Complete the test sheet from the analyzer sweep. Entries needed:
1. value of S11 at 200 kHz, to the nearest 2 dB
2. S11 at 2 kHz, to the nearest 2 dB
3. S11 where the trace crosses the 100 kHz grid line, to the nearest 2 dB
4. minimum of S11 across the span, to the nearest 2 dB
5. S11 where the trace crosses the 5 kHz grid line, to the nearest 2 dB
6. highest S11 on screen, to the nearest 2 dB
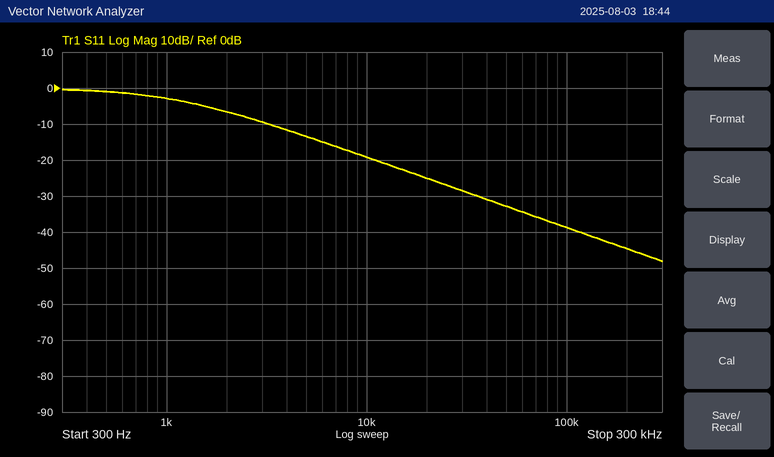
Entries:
-44 dB
-6 dB
-38 dB
-48 dB
-14 dB
0 dB
